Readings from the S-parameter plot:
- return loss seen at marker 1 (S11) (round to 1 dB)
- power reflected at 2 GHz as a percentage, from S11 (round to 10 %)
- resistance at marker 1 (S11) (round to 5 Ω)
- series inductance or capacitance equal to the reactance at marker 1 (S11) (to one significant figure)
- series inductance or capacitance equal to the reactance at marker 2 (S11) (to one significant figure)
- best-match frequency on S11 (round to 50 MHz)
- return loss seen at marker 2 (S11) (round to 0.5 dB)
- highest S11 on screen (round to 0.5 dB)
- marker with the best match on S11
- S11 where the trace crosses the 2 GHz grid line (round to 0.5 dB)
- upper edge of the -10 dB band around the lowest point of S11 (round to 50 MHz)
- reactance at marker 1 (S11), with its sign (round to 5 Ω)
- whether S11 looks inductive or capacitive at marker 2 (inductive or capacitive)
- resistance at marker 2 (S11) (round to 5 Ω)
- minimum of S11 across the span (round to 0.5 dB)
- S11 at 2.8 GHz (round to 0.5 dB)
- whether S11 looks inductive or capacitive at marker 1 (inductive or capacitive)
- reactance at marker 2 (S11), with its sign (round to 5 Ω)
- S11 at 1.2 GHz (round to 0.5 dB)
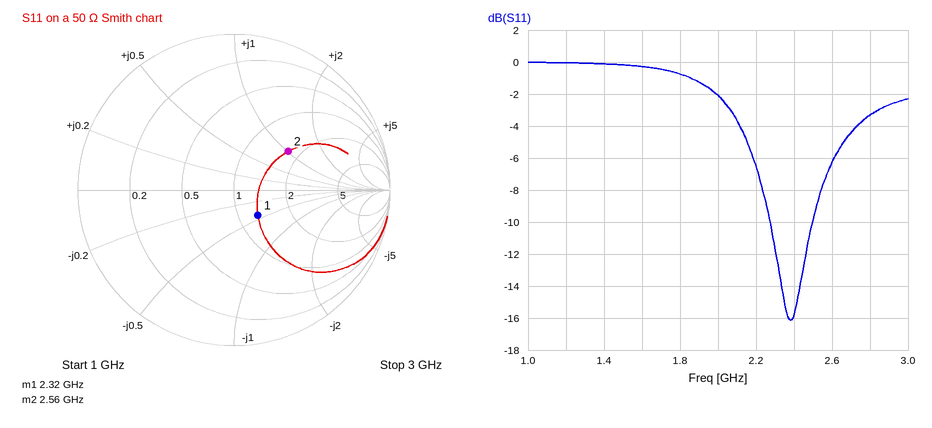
13 dB
60 %
65 Ω
3 pF
3 nH
2.40 GHz
7.5 dB
0.0 dB
marker 1
-2.0 dB
2.50 GHz
-20 Ω
inductive
85 Ω
-16.0 dB
-3.5 dB
capacitive
+50 Ω
0.0 dB
